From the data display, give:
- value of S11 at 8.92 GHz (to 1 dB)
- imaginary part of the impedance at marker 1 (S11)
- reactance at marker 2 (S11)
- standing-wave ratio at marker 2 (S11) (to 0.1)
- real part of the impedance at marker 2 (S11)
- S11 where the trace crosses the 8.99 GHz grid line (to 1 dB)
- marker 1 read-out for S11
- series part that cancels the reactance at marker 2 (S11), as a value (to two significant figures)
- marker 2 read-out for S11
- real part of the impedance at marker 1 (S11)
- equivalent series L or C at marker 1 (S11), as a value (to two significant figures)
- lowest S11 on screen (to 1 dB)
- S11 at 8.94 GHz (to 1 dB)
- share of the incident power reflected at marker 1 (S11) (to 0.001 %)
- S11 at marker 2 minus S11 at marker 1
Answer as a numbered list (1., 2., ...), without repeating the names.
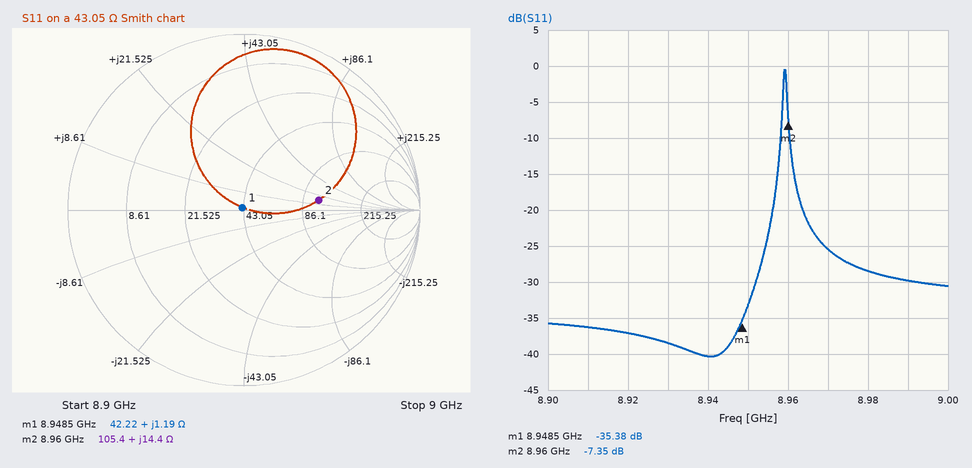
1. -37 dB
2. +1.19 Ω
3. +14.4 Ω
4. 2.5
5. 105.4 Ω
6. -30 dB
7. -35.38 dB
8. 1.2 pF
9. -7.35 dB
10. 42.22 Ω
11. 21 pH
12. -40 dB
13. -40 dB
14. 0.029 %
15. 28.03 dB
